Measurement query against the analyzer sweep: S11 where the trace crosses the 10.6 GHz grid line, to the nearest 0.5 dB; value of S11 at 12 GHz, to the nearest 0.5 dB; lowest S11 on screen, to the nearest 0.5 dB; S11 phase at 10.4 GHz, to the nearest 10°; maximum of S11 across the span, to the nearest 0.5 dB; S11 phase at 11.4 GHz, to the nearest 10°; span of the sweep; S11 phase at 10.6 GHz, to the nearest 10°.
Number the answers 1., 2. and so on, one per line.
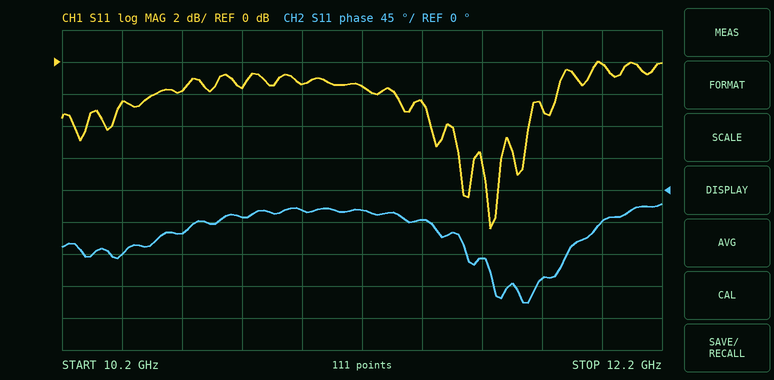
1. -2.0 dB
2. 0.0 dB
3. -10.5 dB
4. -90°
5. 0.0 dB
6. -40°
7. 2 GHz
8. -60°
